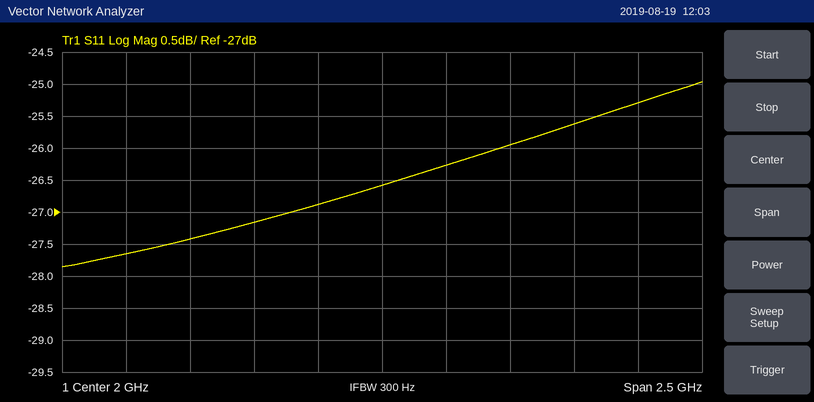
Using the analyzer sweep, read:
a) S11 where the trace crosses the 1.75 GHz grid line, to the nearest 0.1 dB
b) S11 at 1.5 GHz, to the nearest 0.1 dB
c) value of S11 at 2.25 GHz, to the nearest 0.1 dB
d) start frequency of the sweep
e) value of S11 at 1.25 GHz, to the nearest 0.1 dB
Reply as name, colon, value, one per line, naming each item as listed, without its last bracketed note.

S11 where the trace crosses the 1.75 GHz grid line, to the nearest 0.1 dB: -26.9 dB
S11 at 1.5 GHz, to the nearest 0.1 dB: -27.2 dB
value of S11 at 2.25 GHz, to the nearest 0.1 dB: -26.3 dB
start frequency of the sweep: 750 MHz
value of S11 at 1.25 GHz, to the nearest 0.1 dB: -27.4 dB
